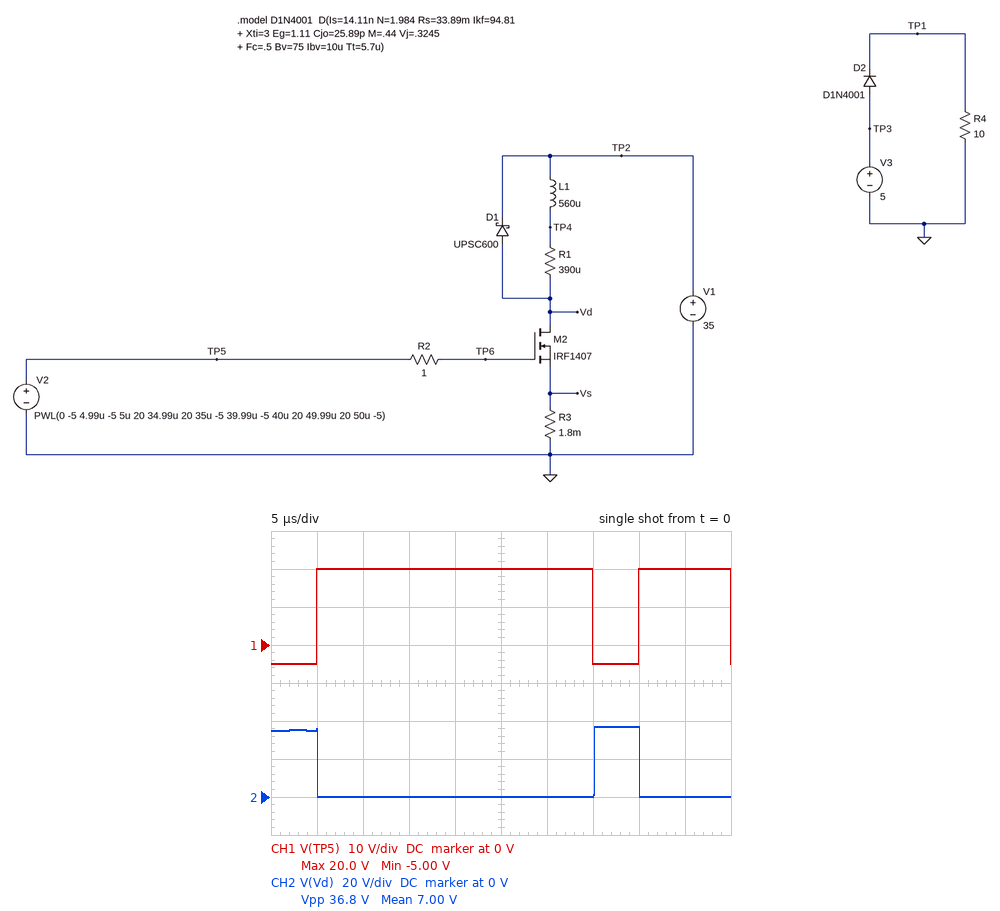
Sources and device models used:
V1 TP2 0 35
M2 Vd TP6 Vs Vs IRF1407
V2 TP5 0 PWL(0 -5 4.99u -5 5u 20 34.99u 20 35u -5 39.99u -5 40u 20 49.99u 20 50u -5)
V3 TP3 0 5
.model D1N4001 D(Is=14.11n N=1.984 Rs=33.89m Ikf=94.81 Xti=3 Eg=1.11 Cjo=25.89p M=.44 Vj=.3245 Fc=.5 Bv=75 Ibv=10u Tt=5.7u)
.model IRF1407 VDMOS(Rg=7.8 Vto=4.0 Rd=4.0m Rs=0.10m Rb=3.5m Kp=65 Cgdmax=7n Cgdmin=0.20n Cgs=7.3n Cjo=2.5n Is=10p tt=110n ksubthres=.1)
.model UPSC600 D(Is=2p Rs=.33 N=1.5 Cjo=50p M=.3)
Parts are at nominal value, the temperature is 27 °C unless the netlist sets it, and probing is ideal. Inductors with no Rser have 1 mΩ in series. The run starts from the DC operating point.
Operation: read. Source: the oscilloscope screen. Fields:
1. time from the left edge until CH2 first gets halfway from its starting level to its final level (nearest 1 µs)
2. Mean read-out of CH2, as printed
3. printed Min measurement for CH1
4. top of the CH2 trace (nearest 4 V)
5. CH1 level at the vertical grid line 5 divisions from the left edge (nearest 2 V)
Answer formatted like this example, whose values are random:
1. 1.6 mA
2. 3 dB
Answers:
1. 5 µs
2. 7.00 V
3. -5.00 V
4. 36 V
5. 20 V
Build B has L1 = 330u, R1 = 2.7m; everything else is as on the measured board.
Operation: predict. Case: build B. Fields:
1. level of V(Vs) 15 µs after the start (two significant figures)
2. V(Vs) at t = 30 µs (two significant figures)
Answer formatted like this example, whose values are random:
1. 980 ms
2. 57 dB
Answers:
1. 1.9 mV
2. 4.8 mV
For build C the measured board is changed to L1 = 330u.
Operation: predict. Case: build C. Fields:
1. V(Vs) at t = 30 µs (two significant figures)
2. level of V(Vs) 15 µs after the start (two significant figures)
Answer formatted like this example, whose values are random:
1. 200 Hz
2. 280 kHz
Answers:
1. 4.8 mV
2. 1.9 mV
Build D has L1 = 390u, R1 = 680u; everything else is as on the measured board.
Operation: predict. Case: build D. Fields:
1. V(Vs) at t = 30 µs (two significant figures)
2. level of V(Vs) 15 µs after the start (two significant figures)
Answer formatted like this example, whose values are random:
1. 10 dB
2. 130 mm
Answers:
1. 4.0 mV
2. 1.6 mV
